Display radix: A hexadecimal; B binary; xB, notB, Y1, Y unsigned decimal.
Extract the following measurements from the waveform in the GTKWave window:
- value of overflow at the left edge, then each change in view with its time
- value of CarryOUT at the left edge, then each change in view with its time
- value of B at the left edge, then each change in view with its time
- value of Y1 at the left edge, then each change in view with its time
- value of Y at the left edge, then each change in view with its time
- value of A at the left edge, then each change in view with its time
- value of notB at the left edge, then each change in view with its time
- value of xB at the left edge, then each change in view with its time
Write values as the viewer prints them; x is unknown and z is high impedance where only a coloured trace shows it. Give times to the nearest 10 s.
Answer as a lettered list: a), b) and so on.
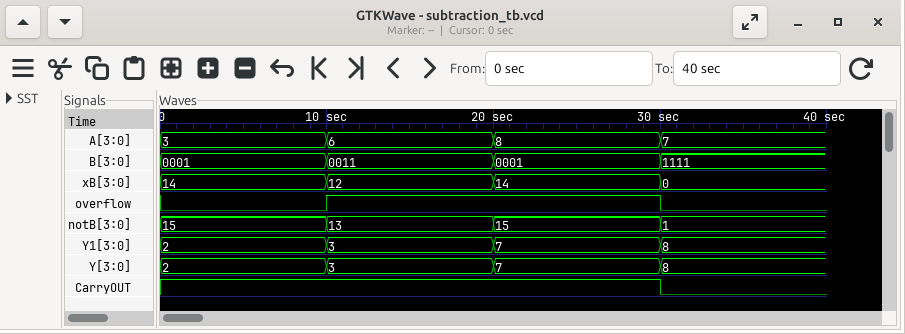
a) 0, 1 at 10 s, 0 at 30 s
b) 1, 0 at 30 s
c) 0001, 0011 at 10 s, 0001 at 20 s, 1111 at 30 s
d) 2, 3 at 10 s, 7 at 20 s, 8 at 30 s
e) 2, 3 at 10 s, 7 at 20 s, 8 at 30 s
f) 3, 6 at 10 s, 8 at 20 s, 7 at 30 s
g) 15, 13 at 10 s, 15 at 20 s, 1 at 30 s
h) 14, 12 at 10 s, 14 at 20 s, 0 at 30 s
